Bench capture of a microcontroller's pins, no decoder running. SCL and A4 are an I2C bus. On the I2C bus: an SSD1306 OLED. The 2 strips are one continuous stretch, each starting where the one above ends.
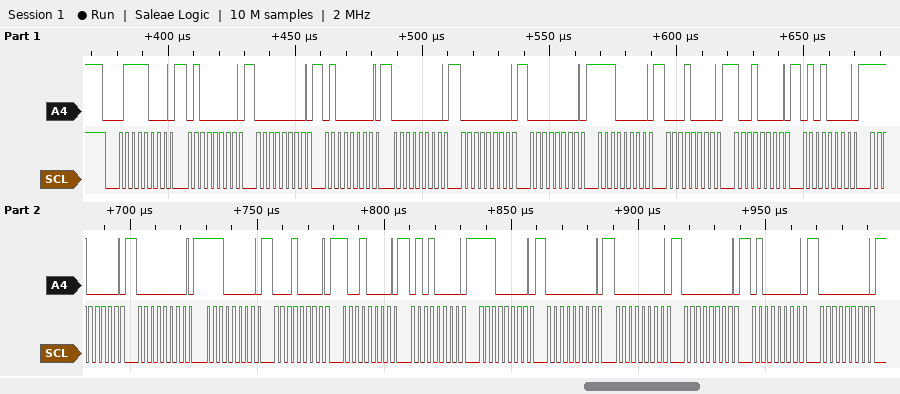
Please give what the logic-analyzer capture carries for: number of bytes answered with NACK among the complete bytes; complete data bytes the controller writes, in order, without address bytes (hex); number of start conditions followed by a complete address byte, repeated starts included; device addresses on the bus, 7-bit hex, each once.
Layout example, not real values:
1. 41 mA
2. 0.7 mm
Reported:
1. 0
2. 40 00 40 00 00 00 E0 10 90 50 E0 00 E0 10 90 50 E0 00 00 00 40 00
3. 1
4. 0x3C
